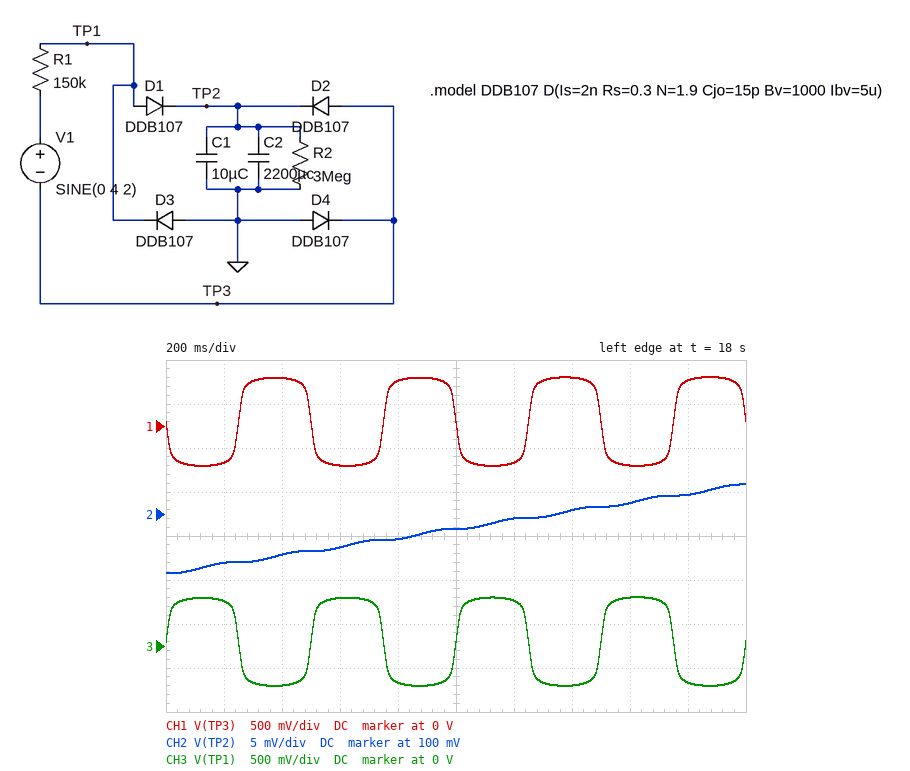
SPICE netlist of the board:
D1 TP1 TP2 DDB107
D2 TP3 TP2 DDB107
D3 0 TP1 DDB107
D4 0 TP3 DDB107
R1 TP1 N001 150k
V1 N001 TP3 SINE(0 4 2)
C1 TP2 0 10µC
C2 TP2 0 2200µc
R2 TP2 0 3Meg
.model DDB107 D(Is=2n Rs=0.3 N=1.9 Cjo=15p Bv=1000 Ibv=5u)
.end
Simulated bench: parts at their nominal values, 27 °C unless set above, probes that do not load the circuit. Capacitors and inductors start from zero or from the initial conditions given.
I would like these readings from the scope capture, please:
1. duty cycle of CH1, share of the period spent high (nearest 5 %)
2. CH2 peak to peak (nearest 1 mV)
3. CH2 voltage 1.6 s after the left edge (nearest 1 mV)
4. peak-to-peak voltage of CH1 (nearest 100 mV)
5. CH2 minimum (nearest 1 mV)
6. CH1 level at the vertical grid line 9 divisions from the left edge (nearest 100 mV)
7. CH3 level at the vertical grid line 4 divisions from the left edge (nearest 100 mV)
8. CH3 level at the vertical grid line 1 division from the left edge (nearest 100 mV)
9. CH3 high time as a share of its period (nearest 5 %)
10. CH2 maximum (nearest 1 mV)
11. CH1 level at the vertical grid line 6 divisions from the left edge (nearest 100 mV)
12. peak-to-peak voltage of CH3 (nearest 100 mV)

50 %
10 mV
101 mV
1.0 V
93 mV
500 mV
-400 mV
500 mV
50 %
103 mV
-400 mV
1.0 V
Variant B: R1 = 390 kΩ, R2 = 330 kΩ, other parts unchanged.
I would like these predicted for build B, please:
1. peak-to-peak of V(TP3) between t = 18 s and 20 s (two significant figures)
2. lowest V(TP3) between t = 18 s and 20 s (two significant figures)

860 mV
-410 mV
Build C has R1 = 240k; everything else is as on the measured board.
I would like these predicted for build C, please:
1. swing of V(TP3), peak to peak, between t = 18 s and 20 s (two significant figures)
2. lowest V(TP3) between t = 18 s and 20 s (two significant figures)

930 mV
-430 mV
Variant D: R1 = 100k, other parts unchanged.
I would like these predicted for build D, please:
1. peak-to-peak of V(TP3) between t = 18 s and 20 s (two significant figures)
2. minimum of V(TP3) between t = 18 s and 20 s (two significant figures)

1.1 V
-470 mV
